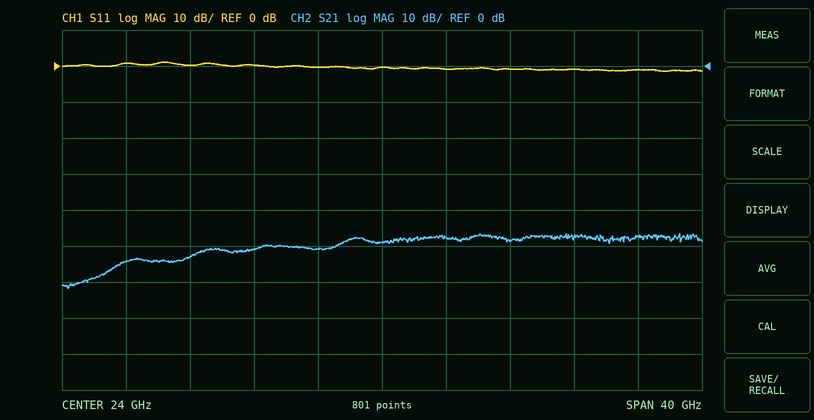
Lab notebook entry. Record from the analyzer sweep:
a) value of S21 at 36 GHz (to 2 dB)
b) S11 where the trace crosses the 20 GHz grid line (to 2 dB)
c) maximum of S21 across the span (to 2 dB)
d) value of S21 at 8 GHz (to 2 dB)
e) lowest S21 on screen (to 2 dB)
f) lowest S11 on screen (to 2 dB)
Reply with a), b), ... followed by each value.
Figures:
a) -48 dB
b) 0 dB
c) -46 dB
d) -54 dB
e) -62 dB
f) -2 dB
